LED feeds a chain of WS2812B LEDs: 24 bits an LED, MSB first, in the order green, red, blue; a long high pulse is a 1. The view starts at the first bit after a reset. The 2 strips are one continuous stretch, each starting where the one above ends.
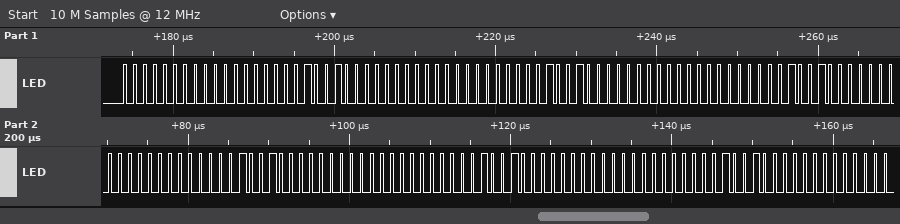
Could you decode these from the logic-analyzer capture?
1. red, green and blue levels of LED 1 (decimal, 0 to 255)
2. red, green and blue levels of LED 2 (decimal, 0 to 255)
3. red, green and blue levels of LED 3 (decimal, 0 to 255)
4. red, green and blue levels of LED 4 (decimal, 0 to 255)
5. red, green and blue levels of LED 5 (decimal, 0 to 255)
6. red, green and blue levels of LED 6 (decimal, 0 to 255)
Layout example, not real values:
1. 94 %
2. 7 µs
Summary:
1. 0, 0, 36
2. 0, 0, 36
3. 0, 0, 36
4. 0, 0, 36
5. 0, 0, 36
6. 0, 0, 36
